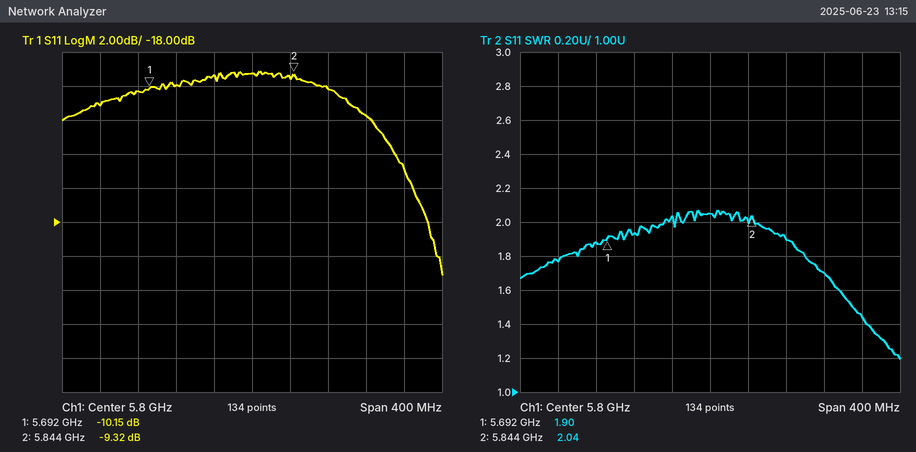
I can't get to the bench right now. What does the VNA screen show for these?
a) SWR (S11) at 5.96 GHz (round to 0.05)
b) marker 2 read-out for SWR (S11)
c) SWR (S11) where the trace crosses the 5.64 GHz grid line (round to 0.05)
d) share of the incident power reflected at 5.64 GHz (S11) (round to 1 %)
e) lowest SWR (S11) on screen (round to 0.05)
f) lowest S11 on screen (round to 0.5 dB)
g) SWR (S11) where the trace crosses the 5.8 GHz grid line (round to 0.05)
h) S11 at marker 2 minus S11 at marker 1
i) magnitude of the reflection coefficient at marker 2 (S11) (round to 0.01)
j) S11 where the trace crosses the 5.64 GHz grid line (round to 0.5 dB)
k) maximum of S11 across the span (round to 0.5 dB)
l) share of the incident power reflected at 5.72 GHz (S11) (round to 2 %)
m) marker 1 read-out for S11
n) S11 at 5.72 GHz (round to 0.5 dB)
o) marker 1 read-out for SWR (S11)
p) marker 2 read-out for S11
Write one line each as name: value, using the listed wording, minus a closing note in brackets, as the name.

SWR (S11) at 5.96 GHz: 1.45
marker 2 read-out for SWR: 2.04
SWR (S11) where the trace crosses the 5.64 GHz grid line: 1.75
share of the incident power reflected at 5.64 GHz (S11): 8 %
lowest SWR (S11) on screen: 1.20
lowest S11 on screen: -21.0 dB
SWR (S11) where the trace crosses the 5.8 GHz grid line: 2.05
S11 at marker 2 minus S11 at marker 1: 0.83 dB
magnitude of the reflection coefficient at marker 2 (S11): 0.34
S11 where the trace crosses the 5.64 GHz grid line: -11.0 dB
maximum of S11 across the span: -9.0 dB
share of the incident power reflected at 5.72 GHz (S11): 10 %
marker 1 read-out for S11: -10.15 dB
S11 at 5.72 GHz: -10.0 dB
marker 1 read-out for SWR: 1.90
marker 2 read-out for S11: -9.32 dB
